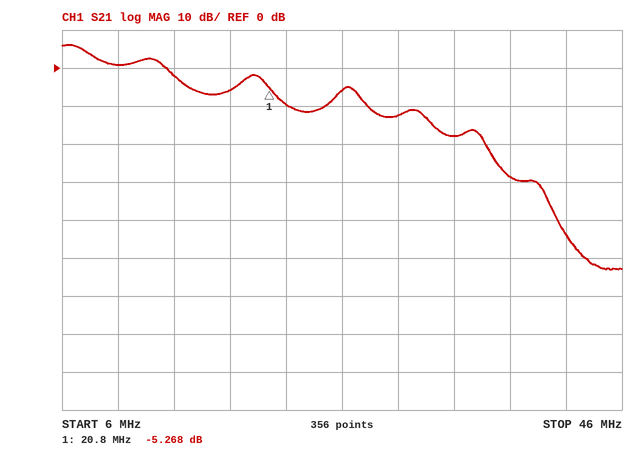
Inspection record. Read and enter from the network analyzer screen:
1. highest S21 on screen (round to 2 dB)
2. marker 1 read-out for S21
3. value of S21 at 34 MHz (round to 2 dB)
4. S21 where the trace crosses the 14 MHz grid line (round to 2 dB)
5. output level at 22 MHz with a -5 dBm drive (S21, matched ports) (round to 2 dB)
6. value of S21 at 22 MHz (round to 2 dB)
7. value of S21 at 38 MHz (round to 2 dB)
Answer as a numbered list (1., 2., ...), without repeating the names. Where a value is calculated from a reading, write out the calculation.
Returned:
1. 6 dB
2. -5.268 dB
3. -18 dB
4. -2 dB
5. -5 dBm + (-10 dB) = -14 dBm
6. -10 dB
7. -28 dB
